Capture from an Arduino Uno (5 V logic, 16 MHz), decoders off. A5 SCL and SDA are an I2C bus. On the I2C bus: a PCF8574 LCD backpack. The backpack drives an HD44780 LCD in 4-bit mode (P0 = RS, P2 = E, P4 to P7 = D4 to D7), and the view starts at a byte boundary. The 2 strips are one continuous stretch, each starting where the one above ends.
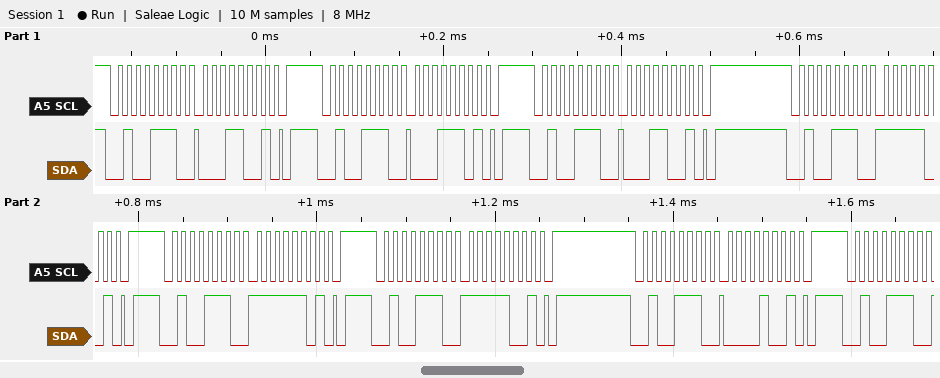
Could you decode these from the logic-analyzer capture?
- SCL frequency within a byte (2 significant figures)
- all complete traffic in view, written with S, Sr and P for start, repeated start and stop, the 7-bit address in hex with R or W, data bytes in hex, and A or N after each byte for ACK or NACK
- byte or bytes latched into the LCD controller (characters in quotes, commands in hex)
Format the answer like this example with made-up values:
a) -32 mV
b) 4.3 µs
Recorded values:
a) 100 kHz
b) S 27W A 19 A P S 27W A 1D A P S 27W A 19 A P S 27W A F9 A P S 27W A FD A P S 27W A F9 A P S 27W A 09 A P S 27W A
c) data 0x1F
